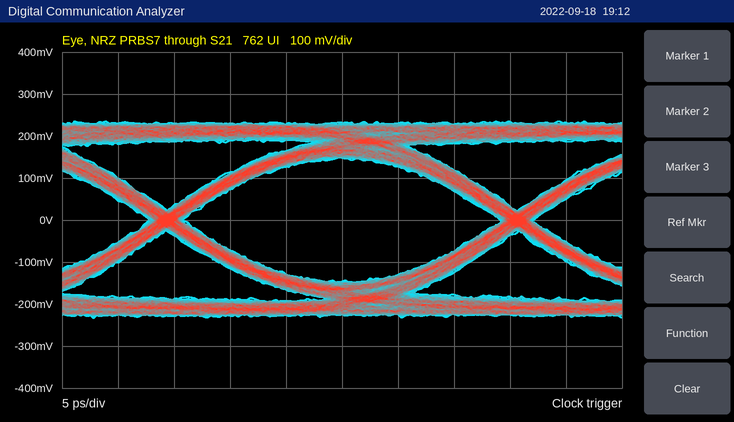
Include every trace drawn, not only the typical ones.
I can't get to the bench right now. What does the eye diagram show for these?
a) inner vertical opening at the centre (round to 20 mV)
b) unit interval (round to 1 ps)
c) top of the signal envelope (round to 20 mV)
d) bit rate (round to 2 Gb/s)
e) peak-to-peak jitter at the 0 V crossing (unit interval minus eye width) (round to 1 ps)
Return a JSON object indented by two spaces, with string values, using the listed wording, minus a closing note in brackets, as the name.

{
  "inner vertical opening at the centre": "300 mV",
  "unit interval": "31 ps",
  "top of the signal envelope": "240 mV",
  "bit rate": "32 Gb/s",
  "peak-to-peak jitter at the 0 V crossing (unit interval minus eye width)": "3 ps"
}
